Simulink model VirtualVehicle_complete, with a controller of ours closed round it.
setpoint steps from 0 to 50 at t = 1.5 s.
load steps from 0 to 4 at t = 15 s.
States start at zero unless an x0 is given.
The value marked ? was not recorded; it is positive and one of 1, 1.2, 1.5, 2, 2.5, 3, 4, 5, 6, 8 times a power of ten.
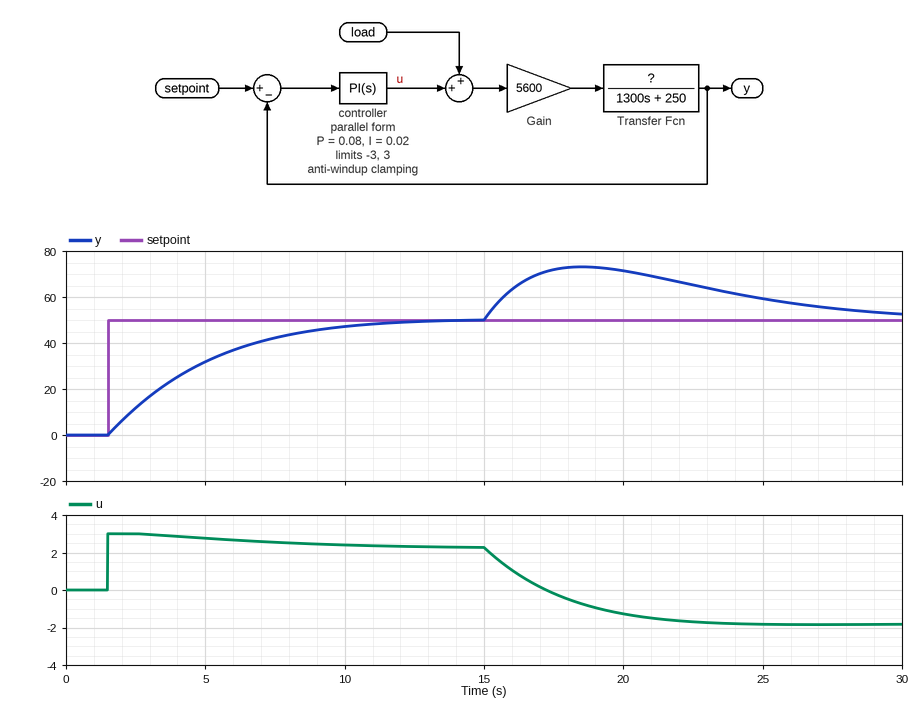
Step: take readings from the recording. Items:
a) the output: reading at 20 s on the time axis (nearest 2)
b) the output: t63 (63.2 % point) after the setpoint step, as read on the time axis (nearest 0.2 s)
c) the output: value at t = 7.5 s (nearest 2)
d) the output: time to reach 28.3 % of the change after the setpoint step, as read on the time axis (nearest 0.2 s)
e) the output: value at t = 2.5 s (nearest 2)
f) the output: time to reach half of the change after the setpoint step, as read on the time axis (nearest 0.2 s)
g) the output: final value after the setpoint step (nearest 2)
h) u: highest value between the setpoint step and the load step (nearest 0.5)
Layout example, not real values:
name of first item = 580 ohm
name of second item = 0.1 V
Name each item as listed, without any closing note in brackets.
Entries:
the output: reading at 20 s on the time axis = 72
the output: t63 (63.2 % point) after the setpoint step, as read on the time axis = 5.0 s
the output: value at t = 7.5 s = 42
the output: time to reach 28.3 % of the change after the setpoint step, as read on the time axis = 2.8 s
the output: value at t = 2.5 s = 12
the output: time to reach half of the change after the setpoint step, as read on the time axis = 4.0 s
the output: final value after the setpoint step = 50
u: highest value between the setpoint step and the load step = 3.0
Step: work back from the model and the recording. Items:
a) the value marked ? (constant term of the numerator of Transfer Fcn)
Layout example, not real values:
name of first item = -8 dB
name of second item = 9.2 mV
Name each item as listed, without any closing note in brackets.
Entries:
the value marked ? = 1
